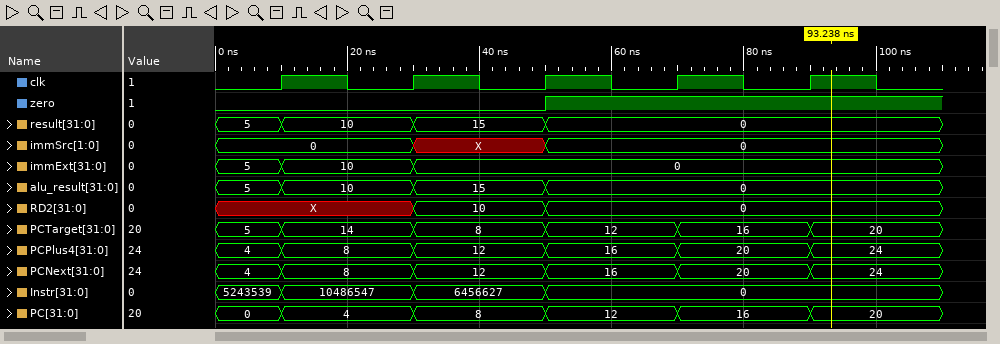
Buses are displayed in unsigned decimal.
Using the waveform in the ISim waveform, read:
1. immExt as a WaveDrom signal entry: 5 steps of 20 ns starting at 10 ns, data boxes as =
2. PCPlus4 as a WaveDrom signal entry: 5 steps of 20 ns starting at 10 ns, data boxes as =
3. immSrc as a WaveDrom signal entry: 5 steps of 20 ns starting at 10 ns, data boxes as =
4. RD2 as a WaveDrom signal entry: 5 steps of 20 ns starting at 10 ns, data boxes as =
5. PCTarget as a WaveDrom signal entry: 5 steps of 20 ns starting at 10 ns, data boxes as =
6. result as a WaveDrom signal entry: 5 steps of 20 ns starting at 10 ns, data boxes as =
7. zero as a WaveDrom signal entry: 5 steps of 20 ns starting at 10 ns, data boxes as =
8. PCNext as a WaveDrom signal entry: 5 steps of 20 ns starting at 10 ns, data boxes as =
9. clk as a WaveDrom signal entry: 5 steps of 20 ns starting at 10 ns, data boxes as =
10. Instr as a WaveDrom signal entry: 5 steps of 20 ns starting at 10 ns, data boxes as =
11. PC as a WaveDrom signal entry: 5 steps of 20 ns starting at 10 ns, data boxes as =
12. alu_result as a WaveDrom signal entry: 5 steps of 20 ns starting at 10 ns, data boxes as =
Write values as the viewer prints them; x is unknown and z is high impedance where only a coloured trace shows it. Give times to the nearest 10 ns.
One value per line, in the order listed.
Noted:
{name: 'immExt', wave: '==...', data: '10 0'}
{name: 'PCPlus4', wave: '=====', data: '8 12 16 20 24'}
{name: 'immSrc', wave: '=x=..', data: '0 0'}
{name: 'RD2', wave: 'x==..', data: '10 0'}
{name: 'PCTarget', wave: '=====', data: '14 8 12 16 20'}
{name: 'result', wave: '===..', data: '10 15 0'}
{name: 'zero', wave: '0.1..'}
{name: 'PCNext', wave: '=====', data: '8 12 16 20 24'}
{name: 'clk', wave: 'p....'}
{name: 'Instr', wave: '===..', data: '10486547 6456627 0'}
{name: 'PC', wave: '=====', data: '4 8 12 16 20'}
{name: 'alu_result', wave: '===..', data: '10 15 0'}
